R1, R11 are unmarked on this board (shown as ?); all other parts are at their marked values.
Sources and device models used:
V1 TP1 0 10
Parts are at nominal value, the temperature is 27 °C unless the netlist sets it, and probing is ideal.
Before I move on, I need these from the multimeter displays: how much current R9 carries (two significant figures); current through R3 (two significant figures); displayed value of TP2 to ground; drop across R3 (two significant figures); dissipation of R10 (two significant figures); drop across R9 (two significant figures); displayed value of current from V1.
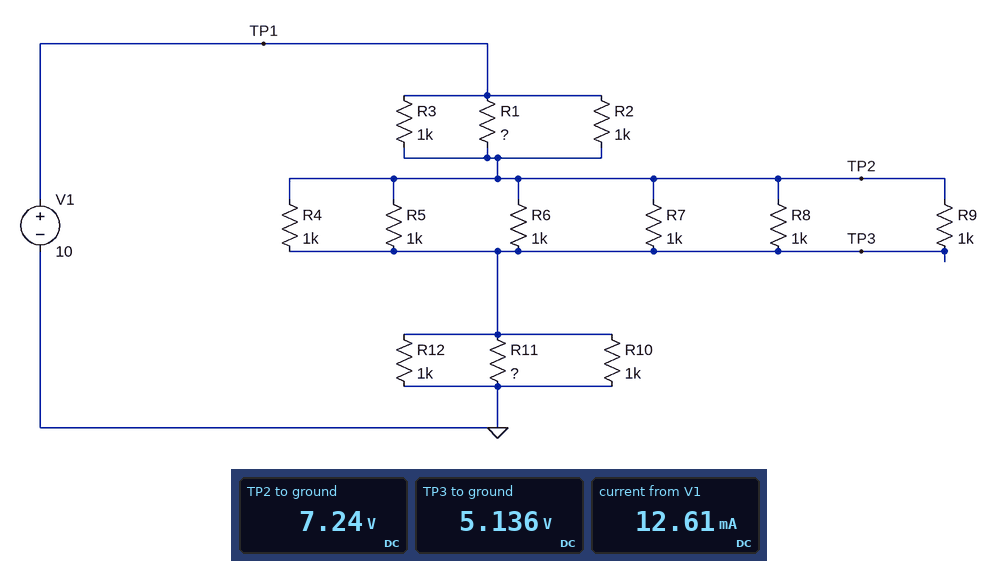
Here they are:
2.1 mA
2.8 mA
7.24 V
2.8 V
26 mW
2.1 V
12.61 mA
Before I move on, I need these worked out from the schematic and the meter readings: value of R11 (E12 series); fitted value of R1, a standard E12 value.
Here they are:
2.2 kΩ
390 Ω
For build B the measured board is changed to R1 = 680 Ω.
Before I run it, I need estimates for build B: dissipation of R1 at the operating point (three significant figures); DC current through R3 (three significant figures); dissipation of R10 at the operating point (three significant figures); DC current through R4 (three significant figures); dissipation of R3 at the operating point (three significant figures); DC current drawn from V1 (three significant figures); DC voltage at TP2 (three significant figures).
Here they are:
16.4 mW
3.34 mA
22.3 mW
1.93 mA
11.2 mW
11.6 mA
6.66 V
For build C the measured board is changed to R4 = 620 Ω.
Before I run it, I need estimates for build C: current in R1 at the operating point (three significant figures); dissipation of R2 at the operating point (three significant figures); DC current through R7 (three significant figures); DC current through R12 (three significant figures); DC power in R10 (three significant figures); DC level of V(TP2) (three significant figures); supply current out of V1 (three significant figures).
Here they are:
7.22 mA
7.94 mW
1.94 mA
5.24 mA
27.4 mW
7.18 V
12.9 mA
